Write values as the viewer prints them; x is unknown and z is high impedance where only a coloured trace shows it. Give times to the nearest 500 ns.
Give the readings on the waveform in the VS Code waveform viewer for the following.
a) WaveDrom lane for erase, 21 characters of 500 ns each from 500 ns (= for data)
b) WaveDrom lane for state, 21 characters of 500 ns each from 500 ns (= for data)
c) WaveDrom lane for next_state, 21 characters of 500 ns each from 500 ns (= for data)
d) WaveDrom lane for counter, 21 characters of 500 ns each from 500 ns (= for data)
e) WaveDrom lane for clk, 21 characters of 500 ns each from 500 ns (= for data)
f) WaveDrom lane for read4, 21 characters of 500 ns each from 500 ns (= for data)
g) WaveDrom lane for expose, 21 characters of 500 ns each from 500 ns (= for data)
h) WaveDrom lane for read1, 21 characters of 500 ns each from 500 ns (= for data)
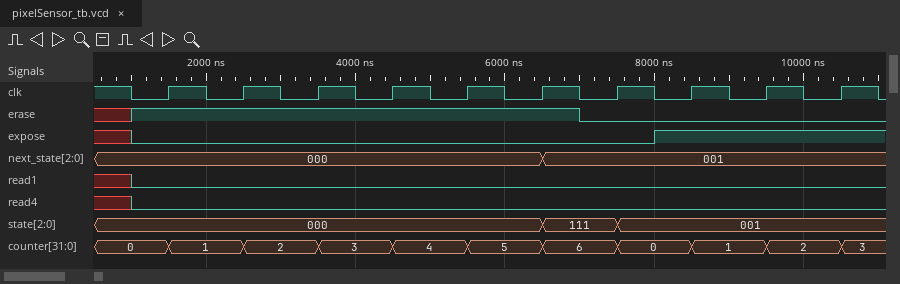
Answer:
{name: 'erase', wave: 'x1...........0.......'}
{name: 'state', wave: '=...........=.=......', data: '000 111 001'}
{name: 'next_state', wave: '=...........=........', data: '000 001'}
{name: 'counter', wave: '=.=.=.=.=.=.=.=.=.=.=', data: '0 1 2 3 4 5 6 0 1 2 3'}
{name: 'clk', wave: '101010101010101010101'}
{name: 'read4', wave: 'x0...................'}
{name: 'expose', wave: 'x0.............1.....'}
{name: 'read1', wave: 'x0...................'}
